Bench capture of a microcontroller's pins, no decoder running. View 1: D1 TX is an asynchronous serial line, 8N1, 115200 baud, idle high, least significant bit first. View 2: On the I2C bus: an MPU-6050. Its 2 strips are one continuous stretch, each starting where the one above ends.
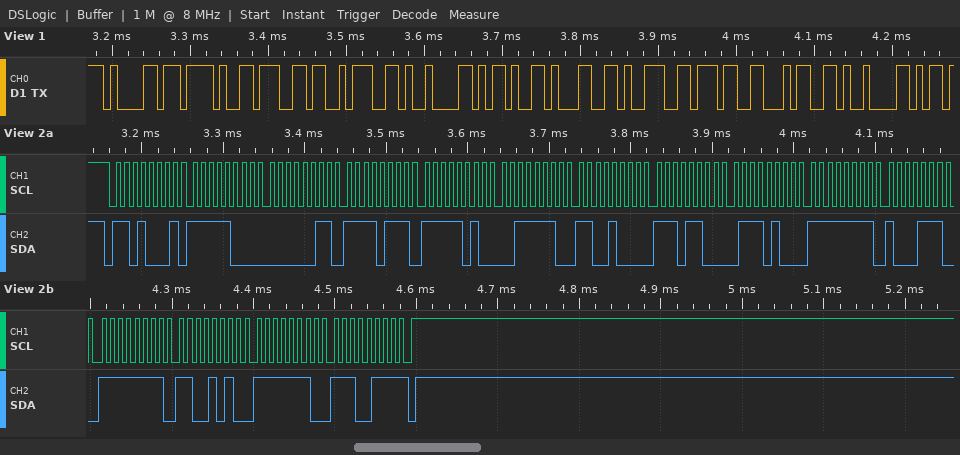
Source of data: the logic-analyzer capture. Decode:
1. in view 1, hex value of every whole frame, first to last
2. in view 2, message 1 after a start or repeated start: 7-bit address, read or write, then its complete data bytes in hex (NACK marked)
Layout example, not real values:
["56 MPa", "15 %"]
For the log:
["61 2F 67 3A 09 2D 31 39 37 34 09", "0x68 read: F8 03 F7 FA 3E C8 EC 74 FF 8E FF CA FE E7 NACK"]
